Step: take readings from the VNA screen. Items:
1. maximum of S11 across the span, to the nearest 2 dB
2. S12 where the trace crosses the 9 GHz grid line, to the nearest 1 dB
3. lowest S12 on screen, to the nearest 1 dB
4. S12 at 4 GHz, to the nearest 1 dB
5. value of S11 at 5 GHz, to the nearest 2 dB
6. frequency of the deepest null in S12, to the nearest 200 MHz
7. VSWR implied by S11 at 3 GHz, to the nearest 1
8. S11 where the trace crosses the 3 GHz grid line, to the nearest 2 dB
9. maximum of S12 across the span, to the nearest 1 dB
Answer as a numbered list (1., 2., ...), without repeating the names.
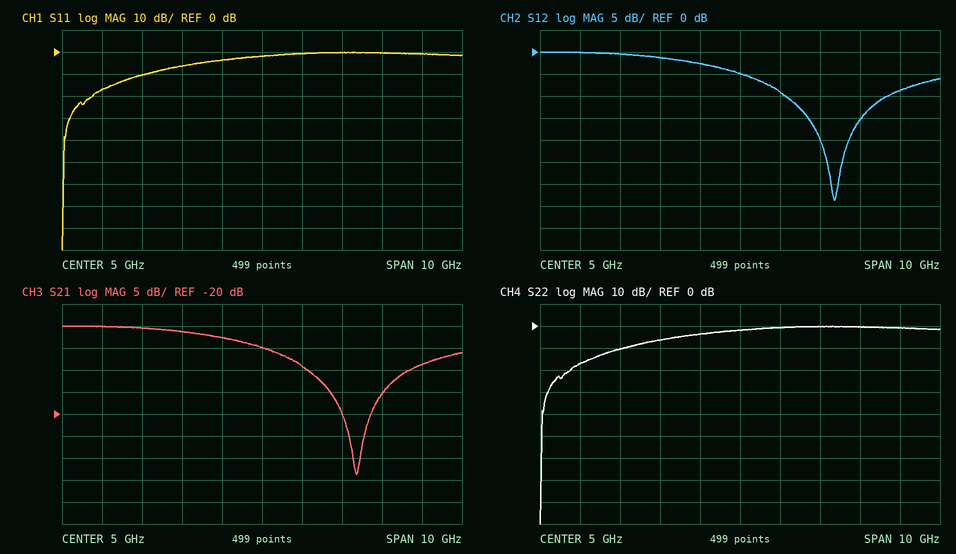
1. 0 dB
2. -9 dB
3. -34 dB
4. -3 dB
5. -2 dB
6. 7.4 GHz
7. 3
8. -6 dB
9. 0 dB
